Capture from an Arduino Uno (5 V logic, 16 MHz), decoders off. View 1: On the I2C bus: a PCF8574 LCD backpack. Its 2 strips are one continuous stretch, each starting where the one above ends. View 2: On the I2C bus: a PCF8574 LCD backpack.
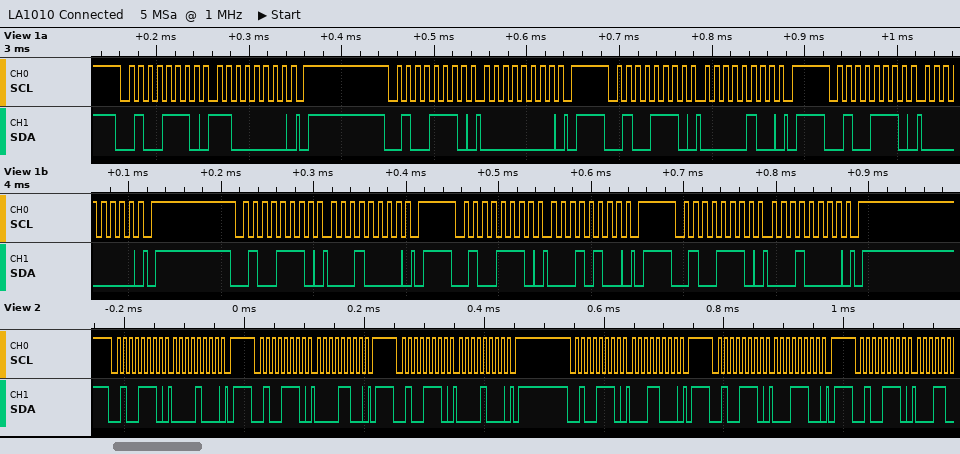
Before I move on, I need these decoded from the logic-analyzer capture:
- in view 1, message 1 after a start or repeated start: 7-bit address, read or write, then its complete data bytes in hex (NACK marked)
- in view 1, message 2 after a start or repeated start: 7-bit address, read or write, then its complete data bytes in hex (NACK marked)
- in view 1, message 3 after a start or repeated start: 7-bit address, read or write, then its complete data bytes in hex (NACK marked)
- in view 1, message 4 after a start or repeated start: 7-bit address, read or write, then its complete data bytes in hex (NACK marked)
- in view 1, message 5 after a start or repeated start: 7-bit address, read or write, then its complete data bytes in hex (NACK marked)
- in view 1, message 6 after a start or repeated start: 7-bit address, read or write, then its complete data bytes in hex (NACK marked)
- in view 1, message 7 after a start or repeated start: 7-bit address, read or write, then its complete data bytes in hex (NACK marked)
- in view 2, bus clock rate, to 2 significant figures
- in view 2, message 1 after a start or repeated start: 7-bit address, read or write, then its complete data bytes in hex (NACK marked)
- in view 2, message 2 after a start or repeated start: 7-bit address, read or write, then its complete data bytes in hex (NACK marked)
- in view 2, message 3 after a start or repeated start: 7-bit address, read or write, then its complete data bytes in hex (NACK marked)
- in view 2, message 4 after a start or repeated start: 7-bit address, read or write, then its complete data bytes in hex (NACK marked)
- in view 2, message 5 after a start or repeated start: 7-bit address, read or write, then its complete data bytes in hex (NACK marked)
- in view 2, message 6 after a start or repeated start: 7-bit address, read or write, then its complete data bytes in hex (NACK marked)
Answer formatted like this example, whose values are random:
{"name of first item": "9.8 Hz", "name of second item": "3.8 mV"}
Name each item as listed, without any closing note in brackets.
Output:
{"in view 1, message 1 after a start or repeated start: 7-bit address, read or write, then its complete data bytes in hex": "0x27 write: C0", "in view 1, message 2 after a start or repeated start: 7-bit address, read or write, then its complete data bytes in hex": "0x27 write: 00", "in view 1, message 3 after a start or repeated start: 7-bit address, read or write, then its complete data bytes in hex": "0x27 write: 04", "in view 1, message 4 after a start or repeated start: 7-bit address, read or write, then its complete data bytes in hex": "0x27 write: 00", "in view 1, message 5 after a start or repeated start: 7-bit address, read or write, then its complete data bytes in hex": "0x27 write: 10", "in view 1, message 6 after a start or repeated start: 7-bit address, read or write, then its complete data bytes in hex": "0x27 write: 14", "in view 1, message 7 after a start or repeated start: 7-bit address, read or write, then its complete data bytes in hex": "0x27 write: 10", "in view 2, bus clock rate, to 2 significant figures": "100 kHz", "in view 2, message 1 after a start or repeated start: 7-bit address, read or write, then its complete data bytes in hex": "0x27 write: 08", "in view 2, message 2 after a start or repeated start: 7-bit address, read or write, then its complete data bytes in hex": "0x27 write: 0C", "in view 2, message 3 after a start or repeated start: 7-bit address, read or write, then its complete data bytes in hex": "0x27 write: 08", "in view 2, message 4 after a start or repeated start: 7-bit address, read or write, then its complete data bytes in hex": "0x27 write: 18", "in view 2, message 5 after a start or repeated start: 7-bit address, read or write, then its complete data bytes in hex": "0x27 write: 1C", "in view 2, message 6 after a start or repeated start: 7-bit address, read or write, then its complete data bytes in hex": "0x27 write"}
